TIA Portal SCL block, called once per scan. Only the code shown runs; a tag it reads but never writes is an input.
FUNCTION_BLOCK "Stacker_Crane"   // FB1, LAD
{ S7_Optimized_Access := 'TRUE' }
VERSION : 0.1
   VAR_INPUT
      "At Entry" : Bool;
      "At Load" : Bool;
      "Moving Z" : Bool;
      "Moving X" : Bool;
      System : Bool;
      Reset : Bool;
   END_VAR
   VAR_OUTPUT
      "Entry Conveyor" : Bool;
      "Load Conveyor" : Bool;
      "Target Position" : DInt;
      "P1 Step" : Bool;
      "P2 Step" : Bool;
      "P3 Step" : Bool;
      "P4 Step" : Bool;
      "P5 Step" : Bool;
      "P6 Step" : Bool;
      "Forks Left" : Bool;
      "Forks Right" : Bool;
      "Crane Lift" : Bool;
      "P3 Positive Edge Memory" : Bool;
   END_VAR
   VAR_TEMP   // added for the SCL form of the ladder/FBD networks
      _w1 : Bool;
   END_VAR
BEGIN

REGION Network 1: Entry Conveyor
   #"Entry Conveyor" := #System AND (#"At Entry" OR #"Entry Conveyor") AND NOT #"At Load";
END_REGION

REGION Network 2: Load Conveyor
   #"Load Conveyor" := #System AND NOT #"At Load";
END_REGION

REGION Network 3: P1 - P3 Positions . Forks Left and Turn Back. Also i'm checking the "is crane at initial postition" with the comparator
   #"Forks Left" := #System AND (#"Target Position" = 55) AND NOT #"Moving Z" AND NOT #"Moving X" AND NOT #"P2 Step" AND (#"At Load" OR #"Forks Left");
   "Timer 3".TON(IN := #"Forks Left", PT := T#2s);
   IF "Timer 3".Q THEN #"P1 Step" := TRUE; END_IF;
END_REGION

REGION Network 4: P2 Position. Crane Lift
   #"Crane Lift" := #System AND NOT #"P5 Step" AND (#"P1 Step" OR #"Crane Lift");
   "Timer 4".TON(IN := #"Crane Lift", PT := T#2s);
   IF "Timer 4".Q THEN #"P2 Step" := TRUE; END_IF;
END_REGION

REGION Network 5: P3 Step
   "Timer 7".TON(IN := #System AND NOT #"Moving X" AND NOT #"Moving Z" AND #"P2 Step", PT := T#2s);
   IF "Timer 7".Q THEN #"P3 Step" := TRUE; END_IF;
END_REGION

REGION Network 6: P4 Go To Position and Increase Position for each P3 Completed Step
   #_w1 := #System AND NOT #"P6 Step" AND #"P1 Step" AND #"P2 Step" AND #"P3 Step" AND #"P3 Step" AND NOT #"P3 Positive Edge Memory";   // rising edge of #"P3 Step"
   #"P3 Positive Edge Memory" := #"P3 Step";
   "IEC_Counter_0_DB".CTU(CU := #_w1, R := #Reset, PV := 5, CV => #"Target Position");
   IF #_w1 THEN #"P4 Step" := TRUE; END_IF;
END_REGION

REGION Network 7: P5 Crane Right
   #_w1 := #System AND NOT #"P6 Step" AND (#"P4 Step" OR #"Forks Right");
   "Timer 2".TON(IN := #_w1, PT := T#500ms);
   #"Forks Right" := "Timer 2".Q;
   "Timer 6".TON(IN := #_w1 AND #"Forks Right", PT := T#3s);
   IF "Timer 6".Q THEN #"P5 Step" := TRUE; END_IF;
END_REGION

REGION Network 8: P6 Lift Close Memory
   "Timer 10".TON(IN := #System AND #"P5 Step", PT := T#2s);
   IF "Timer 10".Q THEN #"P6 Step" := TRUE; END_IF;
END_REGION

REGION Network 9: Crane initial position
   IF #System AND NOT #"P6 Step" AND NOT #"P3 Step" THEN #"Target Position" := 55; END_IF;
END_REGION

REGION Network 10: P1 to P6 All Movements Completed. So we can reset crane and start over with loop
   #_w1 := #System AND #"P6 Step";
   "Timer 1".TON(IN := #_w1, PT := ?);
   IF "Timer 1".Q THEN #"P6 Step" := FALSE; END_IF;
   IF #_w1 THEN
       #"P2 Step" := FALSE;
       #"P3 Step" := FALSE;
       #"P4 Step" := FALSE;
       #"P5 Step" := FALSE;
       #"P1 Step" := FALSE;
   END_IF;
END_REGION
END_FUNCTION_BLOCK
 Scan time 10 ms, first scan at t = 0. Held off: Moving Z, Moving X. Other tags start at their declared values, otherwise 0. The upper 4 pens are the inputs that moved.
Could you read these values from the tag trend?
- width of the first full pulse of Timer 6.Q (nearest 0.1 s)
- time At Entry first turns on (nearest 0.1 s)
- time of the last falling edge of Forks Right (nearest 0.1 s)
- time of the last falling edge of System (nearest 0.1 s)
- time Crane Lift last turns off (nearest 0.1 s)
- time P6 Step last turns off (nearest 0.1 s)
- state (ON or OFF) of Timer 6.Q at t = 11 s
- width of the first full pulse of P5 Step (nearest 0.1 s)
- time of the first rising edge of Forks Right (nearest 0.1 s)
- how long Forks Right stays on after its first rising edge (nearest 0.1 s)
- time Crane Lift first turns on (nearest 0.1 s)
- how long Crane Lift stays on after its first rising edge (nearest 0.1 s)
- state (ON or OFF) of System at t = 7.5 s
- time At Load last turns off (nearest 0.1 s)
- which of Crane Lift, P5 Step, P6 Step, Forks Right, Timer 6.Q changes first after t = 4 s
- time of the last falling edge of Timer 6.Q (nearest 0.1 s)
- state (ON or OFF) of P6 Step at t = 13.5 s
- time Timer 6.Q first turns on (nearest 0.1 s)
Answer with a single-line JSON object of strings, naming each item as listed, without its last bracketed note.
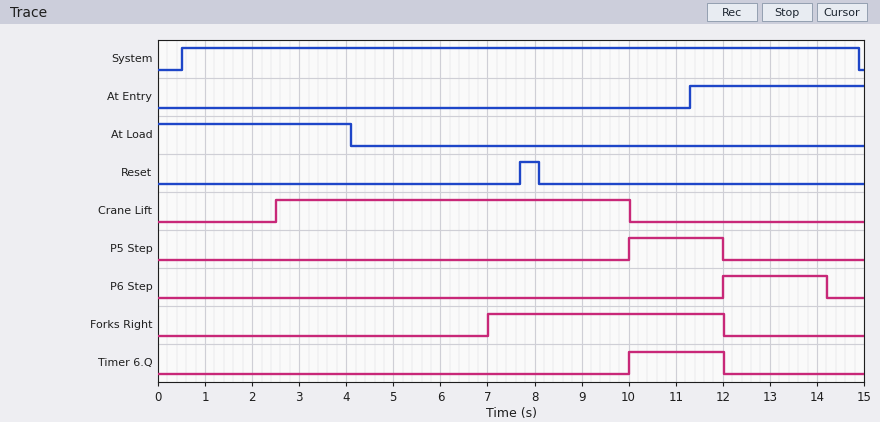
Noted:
{"width of the first full pulse of Timer 6.Q": "2.0 s", "time At Entry first turns on": "11.3 s", "time of the last falling edge of Forks Right": "12.0 s", "time of the last falling edge of System": "14.9 s", "time Crane Lift last turns off": "10.0 s", "time P6 Step last turns off": "14.2 s", "state (ON or OFF) of Timer 6.Q at t = 11 s": "ON", "width of the first full pulse of P5 Step": "2.0 s", "time of the first rising edge of Forks Right": "7.0 s", "how long Forks Right stays on after its first rising edge": "5.0 s", "time Crane Lift first turns on": "2.5 s", "how long Crane Lift stays on after its first rising edge": "7.5 s", "state (ON or OFF) of System at t = 7.5 s": "ON", "time At Load last turns off": "4.1 s", "which of Crane Lift, P5 Step, P6 Step, Forks Right, Timer 6.Q changes first after t = 4 s": "Forks Right", "time of the last falling edge of Timer 6.Q": "12.0 s", "state (ON or OFF) of P6 Step at t = 13.5 s": "ON", "time Timer 6.Q first turns on": "10.0 s"}
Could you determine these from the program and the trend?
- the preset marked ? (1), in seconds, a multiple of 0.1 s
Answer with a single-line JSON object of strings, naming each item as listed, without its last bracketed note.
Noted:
{"the preset marked ? (1), in seconds, a multiple of 0.1 s": "2.2 s"}
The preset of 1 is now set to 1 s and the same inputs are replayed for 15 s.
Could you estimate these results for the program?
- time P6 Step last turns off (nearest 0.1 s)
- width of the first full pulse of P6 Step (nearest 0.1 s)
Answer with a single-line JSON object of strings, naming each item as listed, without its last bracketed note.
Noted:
{"time P6 Step last turns off": "13.0 s", "width of the first full pulse of P6 Step": "1.0 s"}
